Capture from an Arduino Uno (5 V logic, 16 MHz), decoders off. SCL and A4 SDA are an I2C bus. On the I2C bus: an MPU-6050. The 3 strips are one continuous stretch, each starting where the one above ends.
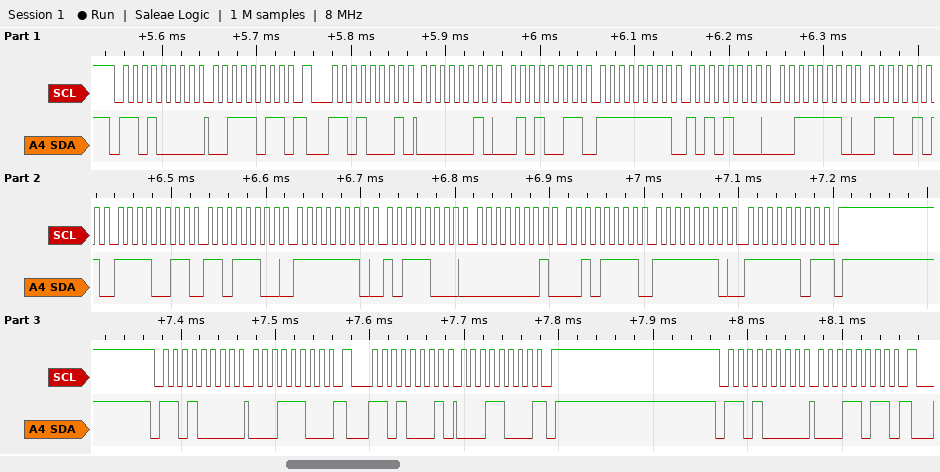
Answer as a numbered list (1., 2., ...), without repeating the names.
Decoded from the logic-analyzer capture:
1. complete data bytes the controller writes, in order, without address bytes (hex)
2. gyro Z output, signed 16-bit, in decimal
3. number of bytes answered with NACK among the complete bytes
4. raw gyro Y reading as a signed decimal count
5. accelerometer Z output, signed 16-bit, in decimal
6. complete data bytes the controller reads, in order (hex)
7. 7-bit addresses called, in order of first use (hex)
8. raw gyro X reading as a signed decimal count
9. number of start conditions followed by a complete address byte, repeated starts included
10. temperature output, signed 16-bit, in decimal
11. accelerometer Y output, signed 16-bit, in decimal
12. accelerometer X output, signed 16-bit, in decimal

1. 3B 1C 1B
2. -259
3. 2
4. 303
5. 15973
6. 02 53 FF A8 3E 65 F3 DC FE B8 01 2F FE FD 18
7. 0x68
8. -328
9. 5
10. -3108
11. -88
12. 595
